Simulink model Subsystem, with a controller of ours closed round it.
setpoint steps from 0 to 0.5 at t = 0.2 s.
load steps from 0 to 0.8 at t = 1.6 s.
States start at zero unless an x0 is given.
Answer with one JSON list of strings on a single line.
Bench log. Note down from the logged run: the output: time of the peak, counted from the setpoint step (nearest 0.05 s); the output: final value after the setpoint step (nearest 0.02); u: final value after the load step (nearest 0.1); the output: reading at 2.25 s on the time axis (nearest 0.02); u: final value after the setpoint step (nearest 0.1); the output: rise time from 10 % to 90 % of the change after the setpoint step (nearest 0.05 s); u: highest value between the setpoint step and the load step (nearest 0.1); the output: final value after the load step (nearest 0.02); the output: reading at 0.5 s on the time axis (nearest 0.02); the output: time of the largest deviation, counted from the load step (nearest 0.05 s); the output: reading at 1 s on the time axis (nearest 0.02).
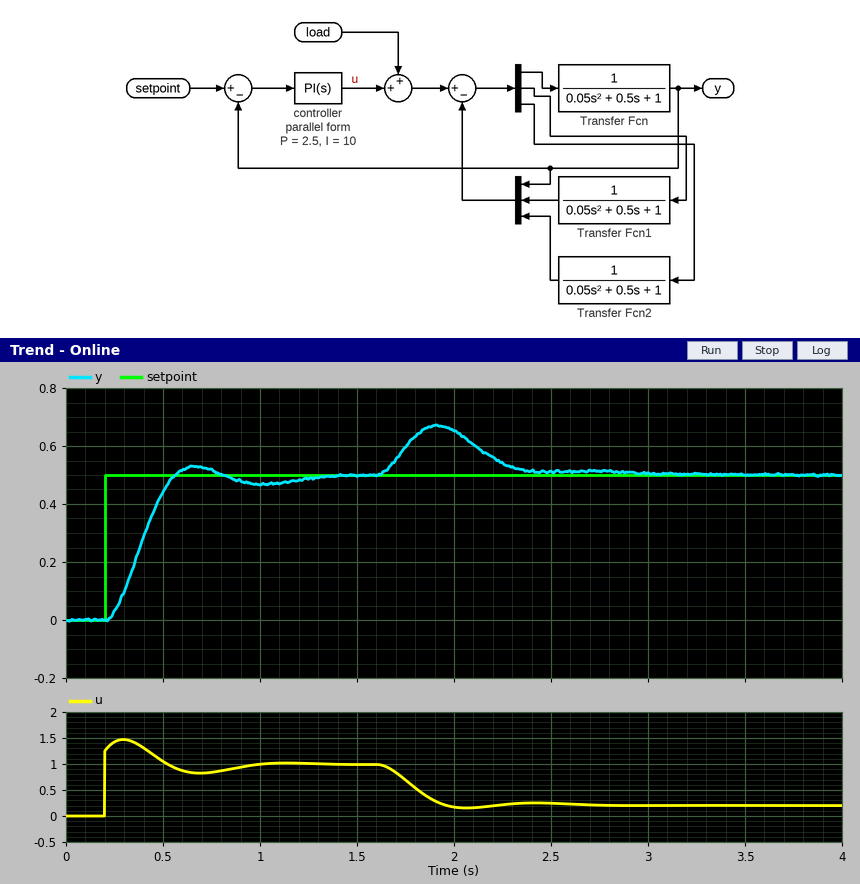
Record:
["0.45 s", "0.50", "0.2", "0.54", "1.0", "0.25 s", "1.5", "0.50", "0.44", "0.30 s", "0.46"]
